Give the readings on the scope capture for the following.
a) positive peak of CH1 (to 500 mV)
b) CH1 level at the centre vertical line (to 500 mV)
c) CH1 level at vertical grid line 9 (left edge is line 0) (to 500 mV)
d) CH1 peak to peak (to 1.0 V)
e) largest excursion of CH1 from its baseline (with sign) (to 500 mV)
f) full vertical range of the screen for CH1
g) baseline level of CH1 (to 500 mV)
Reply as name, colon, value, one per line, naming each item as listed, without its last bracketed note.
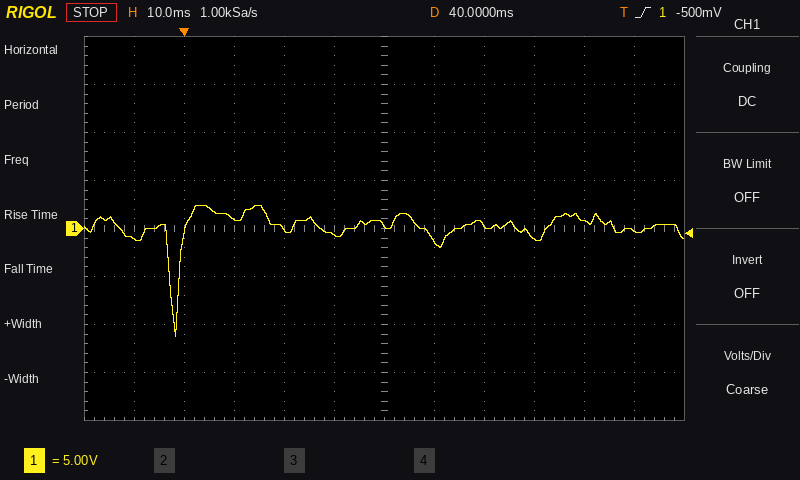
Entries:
positive peak of CH1: 2.5 V
CH1 level at the centre vertical line: 500 mV
CH1 level at vertical grid line 9 (left edge is line 0): -1.0 V
CH1 peak to peak: 14.0 V
largest excursion of CH1 from its baseline (with sign): -11.5 V
full vertical range of the screen for CH1: 40 V
baseline level of CH1: 500 mV
